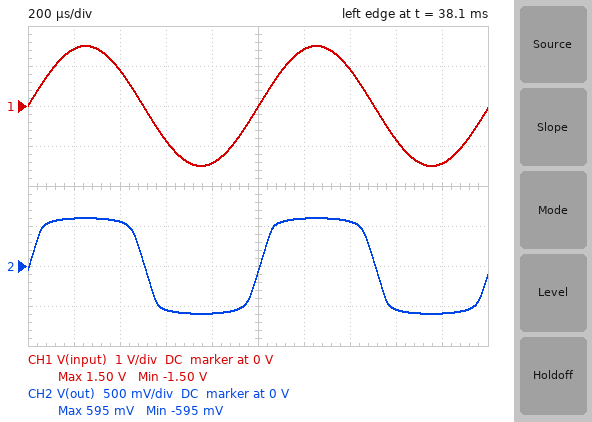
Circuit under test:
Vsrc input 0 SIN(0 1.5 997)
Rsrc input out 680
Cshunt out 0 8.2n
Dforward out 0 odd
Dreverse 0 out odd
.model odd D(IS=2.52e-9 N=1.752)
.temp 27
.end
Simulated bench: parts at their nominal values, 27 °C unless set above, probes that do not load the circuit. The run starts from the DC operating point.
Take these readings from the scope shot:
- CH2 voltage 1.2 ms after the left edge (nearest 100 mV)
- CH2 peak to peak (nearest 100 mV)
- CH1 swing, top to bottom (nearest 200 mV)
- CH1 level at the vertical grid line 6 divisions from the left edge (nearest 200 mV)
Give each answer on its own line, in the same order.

600 mV
1.2 V
3.0 V
1.4 V
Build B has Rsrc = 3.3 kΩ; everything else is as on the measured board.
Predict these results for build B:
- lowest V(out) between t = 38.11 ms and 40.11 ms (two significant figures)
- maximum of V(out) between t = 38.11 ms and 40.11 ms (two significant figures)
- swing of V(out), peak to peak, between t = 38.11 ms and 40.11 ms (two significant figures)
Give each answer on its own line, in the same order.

-530 mV
530 mV
1.1 V
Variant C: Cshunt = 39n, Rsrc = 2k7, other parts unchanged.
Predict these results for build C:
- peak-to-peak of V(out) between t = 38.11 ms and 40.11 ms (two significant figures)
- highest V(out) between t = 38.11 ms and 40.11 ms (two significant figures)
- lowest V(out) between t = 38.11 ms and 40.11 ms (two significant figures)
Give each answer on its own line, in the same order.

1.1 V
540 mV
-540 mV
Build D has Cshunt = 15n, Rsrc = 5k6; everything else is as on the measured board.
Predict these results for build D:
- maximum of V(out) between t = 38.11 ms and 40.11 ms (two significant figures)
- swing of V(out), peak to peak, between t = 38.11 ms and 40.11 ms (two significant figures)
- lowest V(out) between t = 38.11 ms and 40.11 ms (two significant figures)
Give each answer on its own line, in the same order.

510 mV
1.0 V
-510 mV
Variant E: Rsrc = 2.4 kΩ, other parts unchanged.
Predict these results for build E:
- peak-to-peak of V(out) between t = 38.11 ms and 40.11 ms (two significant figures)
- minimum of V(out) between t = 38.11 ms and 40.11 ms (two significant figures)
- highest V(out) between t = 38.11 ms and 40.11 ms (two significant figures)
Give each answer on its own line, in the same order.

1.1 V
-540 mV
540 mV
